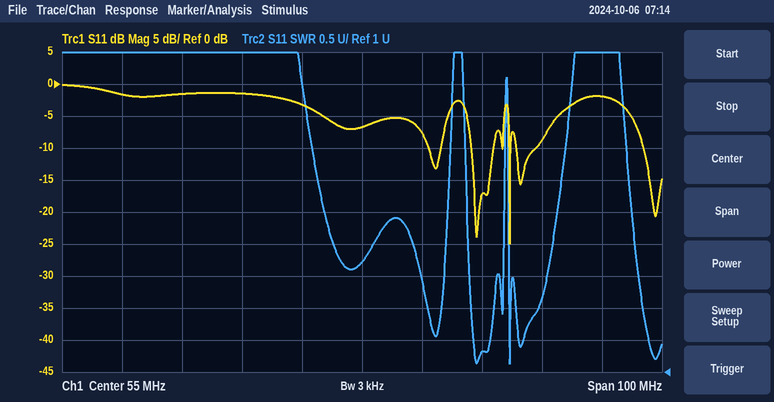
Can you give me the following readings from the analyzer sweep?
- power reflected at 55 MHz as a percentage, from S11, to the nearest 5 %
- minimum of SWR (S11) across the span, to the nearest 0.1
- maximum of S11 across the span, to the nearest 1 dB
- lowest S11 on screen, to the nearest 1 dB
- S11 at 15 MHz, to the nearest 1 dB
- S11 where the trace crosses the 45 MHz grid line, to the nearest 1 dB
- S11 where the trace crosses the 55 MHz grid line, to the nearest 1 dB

20 %
1.1
0 dB
-25 dB
-2 dB
-3 dB
-7 dB
